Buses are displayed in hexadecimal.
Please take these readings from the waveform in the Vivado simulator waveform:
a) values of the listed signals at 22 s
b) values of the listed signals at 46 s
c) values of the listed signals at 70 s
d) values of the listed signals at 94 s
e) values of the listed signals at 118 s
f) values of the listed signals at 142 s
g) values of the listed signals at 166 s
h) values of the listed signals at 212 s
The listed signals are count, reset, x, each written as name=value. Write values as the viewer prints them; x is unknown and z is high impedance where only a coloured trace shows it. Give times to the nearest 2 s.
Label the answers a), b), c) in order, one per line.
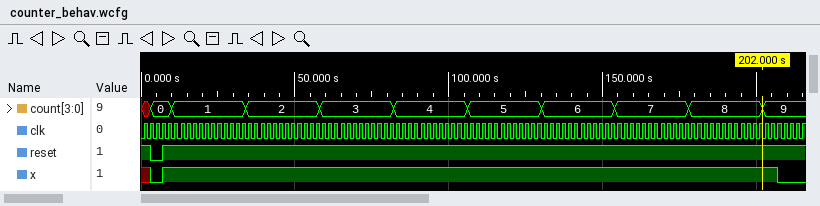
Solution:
a) count=1, reset=1, x=1
b) count=2, reset=1, x=1
c) count=3, reset=1, x=1
d) count=4, reset=1, x=1
e) count=5, reset=1, x=1
f) count=6, reset=1, x=1
g) count=7, reset=1, x=1
h) count=9, reset=1, x=0
